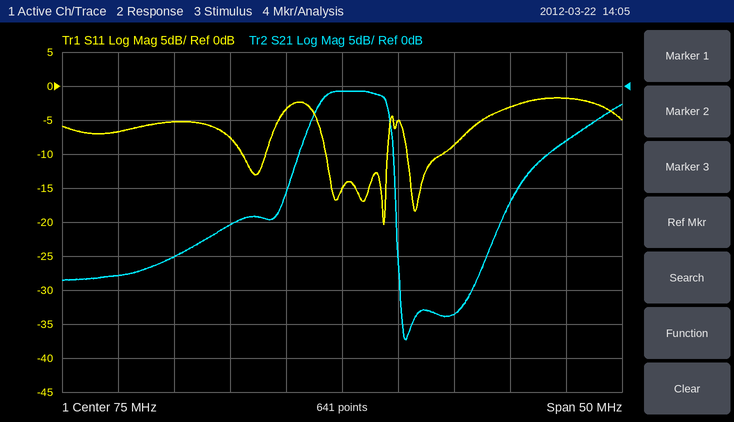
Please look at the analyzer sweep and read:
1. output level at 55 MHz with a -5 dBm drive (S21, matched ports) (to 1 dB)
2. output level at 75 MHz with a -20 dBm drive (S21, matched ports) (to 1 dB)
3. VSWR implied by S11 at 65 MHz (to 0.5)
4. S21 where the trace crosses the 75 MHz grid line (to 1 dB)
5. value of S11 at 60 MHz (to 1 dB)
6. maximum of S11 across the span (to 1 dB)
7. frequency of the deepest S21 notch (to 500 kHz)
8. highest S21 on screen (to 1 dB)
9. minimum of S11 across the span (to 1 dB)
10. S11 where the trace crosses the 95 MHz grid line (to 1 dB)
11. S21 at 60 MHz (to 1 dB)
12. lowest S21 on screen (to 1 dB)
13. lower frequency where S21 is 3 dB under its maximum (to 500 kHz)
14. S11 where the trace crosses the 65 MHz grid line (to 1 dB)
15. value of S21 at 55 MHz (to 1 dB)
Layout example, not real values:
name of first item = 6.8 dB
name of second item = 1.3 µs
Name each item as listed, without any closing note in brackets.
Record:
output level at 55 MHz with a -5 dBm drive (S21, matched ports) = -33 dBm
output level at 75 MHz with a -20 dBm drive (S21, matched ports) = -21 dBm
VSWR implied by S11 at 65 MHz = 2.5
S21 where the trace crosses the 75 MHz grid line = -1 dB
value of S11 at 60 MHz = -5 dB
maximum of S11 across the span = -2 dB
frequency of the deepest S21 notch = 80.5 MHz
highest S21 on screen = -1 dB
minimum of S11 across the span = -20 dB
S11 where the trace crosses the 95 MHz grid line = -2 dB
S21 at 60 MHz = -25 dB
lowest S21 on screen = -37 dB
lower frequency where S21 is 3 dB under its maximum = 72.5 MHz
S11 where the trace crosses the 65 MHz grid line = -8 dB
value of S21 at 55 MHz = -28 dB
